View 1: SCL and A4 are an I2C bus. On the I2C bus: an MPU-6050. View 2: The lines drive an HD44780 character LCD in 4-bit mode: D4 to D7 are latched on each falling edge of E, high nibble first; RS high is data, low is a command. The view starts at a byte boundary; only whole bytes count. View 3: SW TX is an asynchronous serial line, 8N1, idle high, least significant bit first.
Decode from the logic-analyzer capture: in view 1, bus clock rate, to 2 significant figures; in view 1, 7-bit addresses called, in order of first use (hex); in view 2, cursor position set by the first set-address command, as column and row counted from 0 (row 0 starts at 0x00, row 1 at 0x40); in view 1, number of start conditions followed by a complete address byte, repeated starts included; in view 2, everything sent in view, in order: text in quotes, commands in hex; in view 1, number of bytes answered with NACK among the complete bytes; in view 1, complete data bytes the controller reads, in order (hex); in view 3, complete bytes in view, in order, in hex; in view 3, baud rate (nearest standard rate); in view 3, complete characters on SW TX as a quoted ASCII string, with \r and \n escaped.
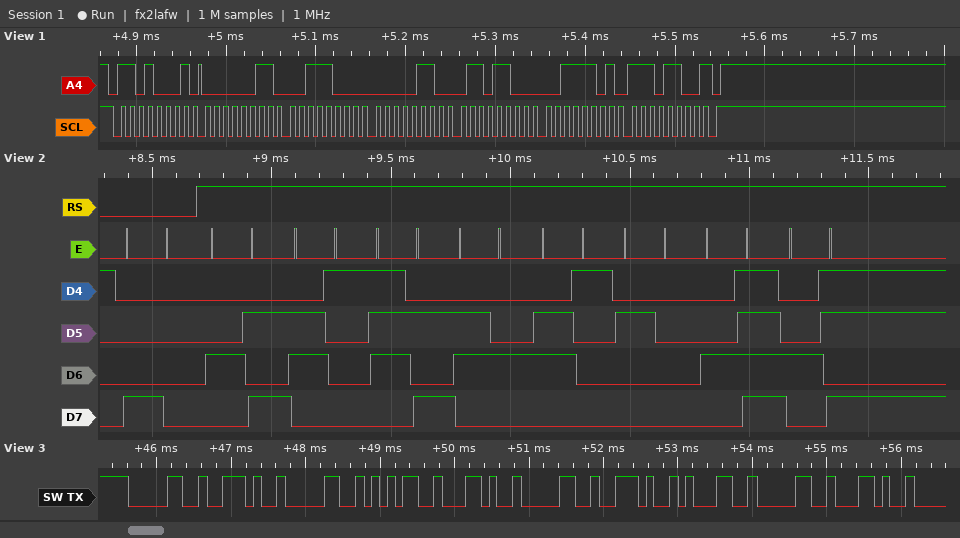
100 kHz
0x68
column 0, row 0
1
0x80 "Jazda OK"
1
03 38 06 6C 3D EC
0x30 0x2E 0x30 0x35 0x2C 0x30 0x2E 0x31 0x30 0x2C
9600 baud
"0.05,0.10,"
